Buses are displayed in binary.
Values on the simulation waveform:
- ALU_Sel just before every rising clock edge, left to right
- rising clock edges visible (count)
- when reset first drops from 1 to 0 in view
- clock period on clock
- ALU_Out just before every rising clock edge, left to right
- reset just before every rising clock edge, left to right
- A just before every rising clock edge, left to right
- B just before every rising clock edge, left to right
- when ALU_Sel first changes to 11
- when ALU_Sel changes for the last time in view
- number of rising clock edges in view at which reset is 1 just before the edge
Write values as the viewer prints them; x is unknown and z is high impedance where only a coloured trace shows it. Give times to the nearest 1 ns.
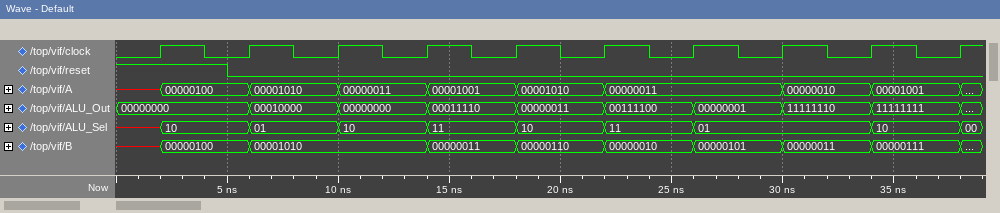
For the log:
x, 10, 01, 10, 11, 10, 11, 01, 01, 10
10
5 ns
4 ns
00000000, 00000000, 00010000, 00000000, 00011110, 00000011, 00111100, 00000001, 11111110, 11111111
1 0 0 0 0 0 0 0 0 0
x, 00000100, 00001010, 00000011, 00001001, 00001010, 00000011, 00000011, 00000010, 00001001
x, 00000100, 00001010, 00001010, 00000011, 00000110, 00000010, 00000101, 00000011, 00000111
14 ns
38 ns
1
